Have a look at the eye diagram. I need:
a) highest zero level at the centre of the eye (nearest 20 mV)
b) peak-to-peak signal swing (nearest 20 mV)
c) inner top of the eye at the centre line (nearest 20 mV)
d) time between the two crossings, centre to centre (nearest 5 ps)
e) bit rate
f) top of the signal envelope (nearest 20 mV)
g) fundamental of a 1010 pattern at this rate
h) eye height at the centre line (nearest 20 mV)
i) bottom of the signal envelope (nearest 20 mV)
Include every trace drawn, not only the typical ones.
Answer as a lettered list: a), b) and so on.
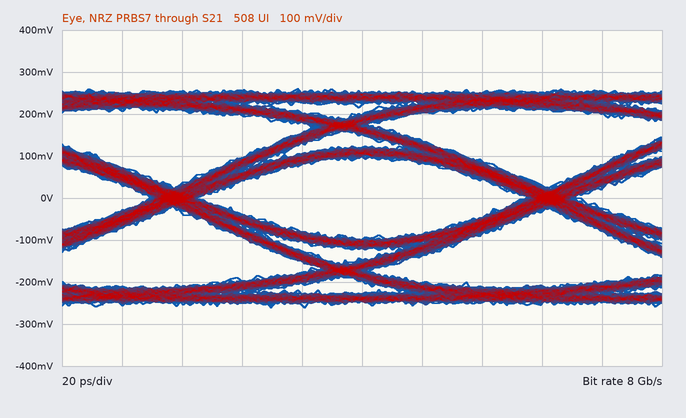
a) -100 mV
b) 520 mV
c) 100 mV
d) 125 ps
e) 8 Gb/s
f) 260 mV
g) 4 GHz
h) 200 mV
i) -260 mV
